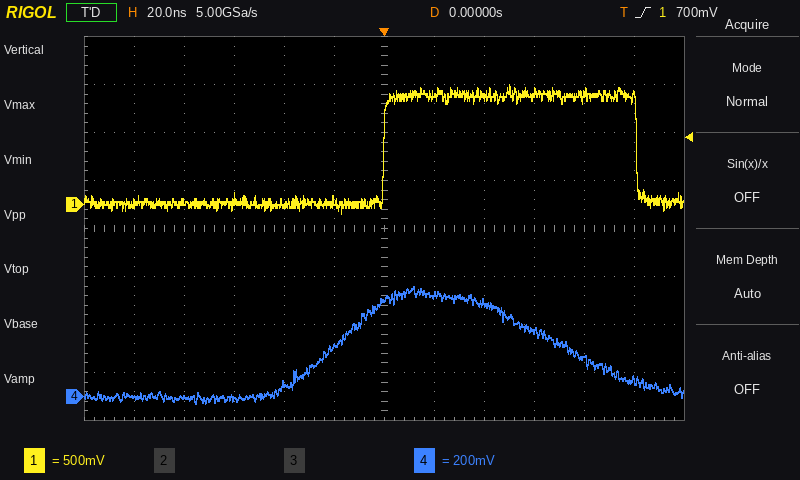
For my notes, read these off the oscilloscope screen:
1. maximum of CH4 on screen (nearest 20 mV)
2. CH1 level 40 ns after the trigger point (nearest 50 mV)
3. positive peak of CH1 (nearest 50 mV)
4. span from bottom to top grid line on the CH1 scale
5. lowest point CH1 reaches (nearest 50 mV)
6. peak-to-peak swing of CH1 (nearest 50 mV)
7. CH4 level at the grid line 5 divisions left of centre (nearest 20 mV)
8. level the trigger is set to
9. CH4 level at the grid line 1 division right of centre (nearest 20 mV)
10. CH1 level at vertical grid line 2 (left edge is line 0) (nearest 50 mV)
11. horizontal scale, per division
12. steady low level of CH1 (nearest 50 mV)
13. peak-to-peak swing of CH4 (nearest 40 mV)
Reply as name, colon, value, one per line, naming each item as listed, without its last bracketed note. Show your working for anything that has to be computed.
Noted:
maximum of CH4 on screen: 460 mV
CH1 level 40 ns after the trigger point: 1.15 V
positive peak of CH1: 1.25 V
span from bottom to top grid line on the CH1 scale: 4 V
lowest point CH1 reaches: -100 mV
peak-to-peak swing of CH1: 1.25 V − (-100 mV) = 1.35 V
CH4 level at the grid line 5 divisions left of centre: 0 mV
level the trigger is set to: 700 mV
CH4 level at the grid line 1 division right of centre: 420 mV
CH1 level at vertical grid line 2 (left edge is line 0): 50 mV
horizontal scale, per division: 20 ns
steady low level of CH1: 0 mV
peak-to-peak swing of CH4: 480 mV
